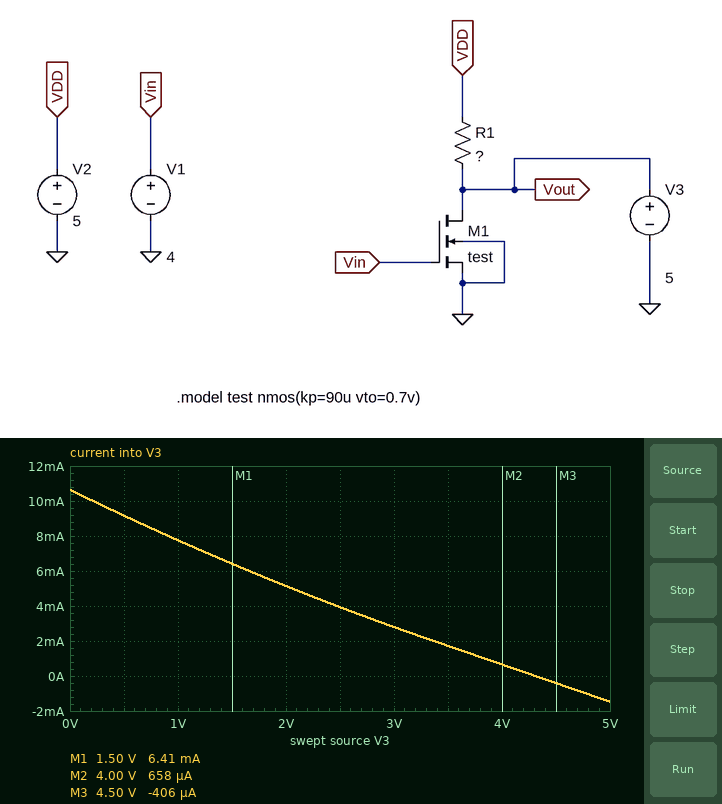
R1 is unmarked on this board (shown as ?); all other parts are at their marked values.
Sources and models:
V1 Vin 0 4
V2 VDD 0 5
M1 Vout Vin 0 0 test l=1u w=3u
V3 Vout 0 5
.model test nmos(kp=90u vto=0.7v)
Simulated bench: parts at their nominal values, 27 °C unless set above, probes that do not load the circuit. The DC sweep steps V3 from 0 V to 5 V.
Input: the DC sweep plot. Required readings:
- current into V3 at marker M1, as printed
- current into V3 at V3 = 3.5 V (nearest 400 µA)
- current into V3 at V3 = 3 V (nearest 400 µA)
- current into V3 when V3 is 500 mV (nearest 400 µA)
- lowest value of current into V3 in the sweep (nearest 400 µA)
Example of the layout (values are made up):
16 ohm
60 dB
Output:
6.41 mA
1.6 mA
2.8 mA
9.2 mA
-1.6 mA
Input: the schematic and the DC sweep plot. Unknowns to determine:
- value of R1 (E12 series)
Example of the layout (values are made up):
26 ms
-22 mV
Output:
470 Ω
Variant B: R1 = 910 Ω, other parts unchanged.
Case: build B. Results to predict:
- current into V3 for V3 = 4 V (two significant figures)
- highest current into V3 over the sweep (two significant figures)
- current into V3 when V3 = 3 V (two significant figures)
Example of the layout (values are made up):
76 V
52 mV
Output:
-370 µA
5.5 mA
740 µA
